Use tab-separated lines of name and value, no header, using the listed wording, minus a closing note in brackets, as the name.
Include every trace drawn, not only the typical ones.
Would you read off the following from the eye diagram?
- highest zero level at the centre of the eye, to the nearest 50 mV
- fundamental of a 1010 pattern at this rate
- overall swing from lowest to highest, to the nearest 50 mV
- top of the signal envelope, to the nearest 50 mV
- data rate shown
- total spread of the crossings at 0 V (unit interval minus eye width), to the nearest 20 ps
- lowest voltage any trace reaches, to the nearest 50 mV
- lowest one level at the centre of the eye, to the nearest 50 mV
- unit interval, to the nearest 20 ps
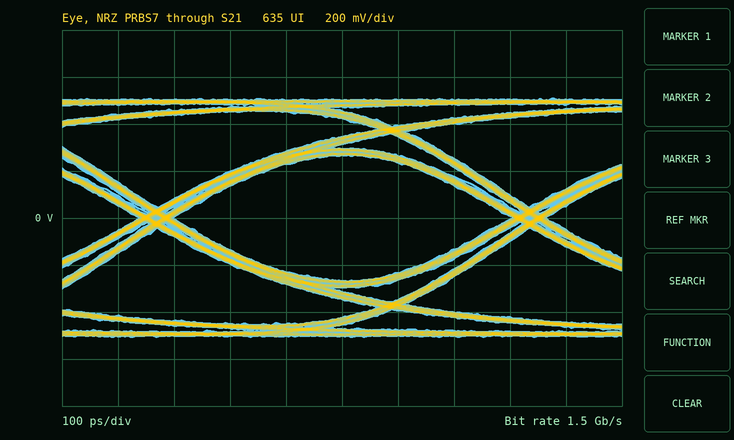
highest zero level at the centre of the eye, to the nearest 50 mV	-250 mV
fundamental of a 1010 pattern at this rate	750 MHz
overall swing from lowest to highest, to the nearest 50 mV	1.00 V
top of the signal envelope, to the nearest 50 mV	500 mV
data rate shown	1.5 Gb/s
total spread of the crossings at 0 V (unit interval minus eye width), to the nearest 20 ps	60 ps
lowest voltage any trace reaches, to the nearest 50 mV	-500 mV
lowest one level at the centre of the eye, to the nearest 50 mV	250 mV
unit interval, to the nearest 20 ps	660 ps
